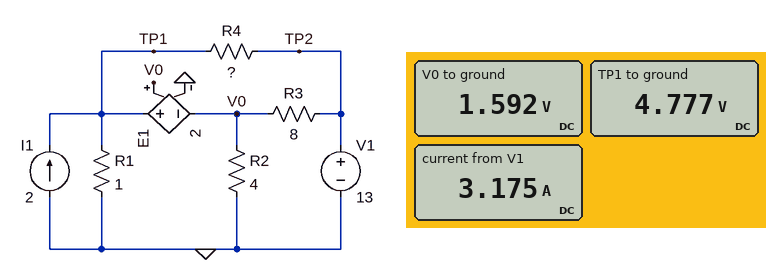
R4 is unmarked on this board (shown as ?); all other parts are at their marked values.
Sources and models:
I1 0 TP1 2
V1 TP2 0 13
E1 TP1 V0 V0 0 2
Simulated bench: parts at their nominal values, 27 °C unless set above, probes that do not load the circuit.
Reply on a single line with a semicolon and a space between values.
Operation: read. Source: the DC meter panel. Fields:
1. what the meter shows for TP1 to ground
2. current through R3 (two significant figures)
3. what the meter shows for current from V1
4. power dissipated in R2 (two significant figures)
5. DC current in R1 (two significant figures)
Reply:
4.777 V; 1.4 A; 3.175 A; 630 mW; 4.8 A
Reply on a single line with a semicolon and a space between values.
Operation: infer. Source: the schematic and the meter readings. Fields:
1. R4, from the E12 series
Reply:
4.7 Ω
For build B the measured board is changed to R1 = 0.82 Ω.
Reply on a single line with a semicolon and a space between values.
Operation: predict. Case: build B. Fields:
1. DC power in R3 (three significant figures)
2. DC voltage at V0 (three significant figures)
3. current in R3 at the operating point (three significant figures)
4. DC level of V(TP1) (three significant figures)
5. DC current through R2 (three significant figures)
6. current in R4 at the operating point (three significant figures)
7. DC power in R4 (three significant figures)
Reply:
16.9 W; 1.37 V; 1.45 A; 4.10 V; 342 mA; 1.89 A; 16.8 W
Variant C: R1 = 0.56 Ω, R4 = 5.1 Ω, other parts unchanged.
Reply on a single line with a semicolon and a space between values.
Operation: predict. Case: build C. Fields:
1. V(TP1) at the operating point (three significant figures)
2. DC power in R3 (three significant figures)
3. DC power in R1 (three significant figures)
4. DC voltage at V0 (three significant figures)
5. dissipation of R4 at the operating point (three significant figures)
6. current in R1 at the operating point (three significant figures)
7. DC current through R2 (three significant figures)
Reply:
2.93 V; 18.1 W; 15.3 W; 977 mV; 19.9 W; 5.23 A; 244 mA
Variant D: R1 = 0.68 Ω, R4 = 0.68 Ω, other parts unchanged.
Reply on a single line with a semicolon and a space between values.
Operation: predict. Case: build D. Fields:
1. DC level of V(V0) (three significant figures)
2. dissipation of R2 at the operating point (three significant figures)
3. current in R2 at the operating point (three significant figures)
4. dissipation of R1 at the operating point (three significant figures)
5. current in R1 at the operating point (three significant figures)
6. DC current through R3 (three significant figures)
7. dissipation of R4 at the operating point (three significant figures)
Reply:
2.47 V; 1.53 W; 618 mA; 80.9 W; 10.9 A; 1.32 A; 45.8 W
